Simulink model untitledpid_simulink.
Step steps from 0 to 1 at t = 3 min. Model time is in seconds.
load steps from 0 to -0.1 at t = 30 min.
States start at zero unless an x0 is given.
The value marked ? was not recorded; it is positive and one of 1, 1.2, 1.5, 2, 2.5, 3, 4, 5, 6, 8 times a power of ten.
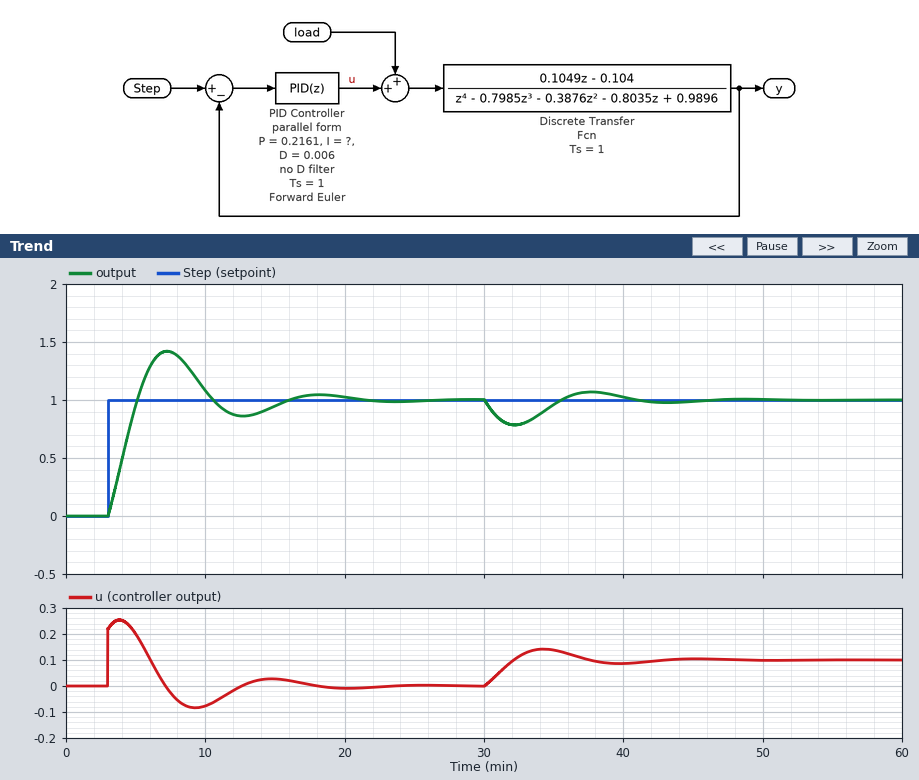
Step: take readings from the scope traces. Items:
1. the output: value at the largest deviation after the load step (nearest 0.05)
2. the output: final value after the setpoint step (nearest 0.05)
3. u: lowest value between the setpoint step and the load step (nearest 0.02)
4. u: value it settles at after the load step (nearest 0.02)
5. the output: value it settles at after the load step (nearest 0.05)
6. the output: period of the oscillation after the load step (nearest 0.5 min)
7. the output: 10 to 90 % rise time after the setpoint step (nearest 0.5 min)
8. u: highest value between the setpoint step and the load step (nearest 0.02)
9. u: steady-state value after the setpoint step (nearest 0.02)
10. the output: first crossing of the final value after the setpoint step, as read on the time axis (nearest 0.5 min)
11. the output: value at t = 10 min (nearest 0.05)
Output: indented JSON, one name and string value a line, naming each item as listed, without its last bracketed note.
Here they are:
{
  "the output: value at the largest deviation after the load step": "0.80",
  "the output: final value after the setpoint step": "1.00",
  "u: lowest value between the setpoint step and the load step": "-0.08",
  "u: value it settles at after the load step": "0.10",
  "the output: value it settles at after the load step": "1.00",
  "the output: period of the oscillation after the load step": "11.0 min",
  "the output: 10 to 90 % rise time after the setpoint step": "1.5 min",
  "u: highest value between the setpoint step and the load step": "0.26",
  "u: steady-state value after the setpoint step": "0.00",
  "the output: first crossing of the final value after the setpoint step, as read on the time axis": "5.0 min",
  "the output: value at t = 10 min": "1.10"
}
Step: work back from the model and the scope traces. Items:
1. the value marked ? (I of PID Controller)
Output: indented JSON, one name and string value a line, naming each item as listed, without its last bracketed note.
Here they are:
{
  "the value marked ?": "0.003"
}
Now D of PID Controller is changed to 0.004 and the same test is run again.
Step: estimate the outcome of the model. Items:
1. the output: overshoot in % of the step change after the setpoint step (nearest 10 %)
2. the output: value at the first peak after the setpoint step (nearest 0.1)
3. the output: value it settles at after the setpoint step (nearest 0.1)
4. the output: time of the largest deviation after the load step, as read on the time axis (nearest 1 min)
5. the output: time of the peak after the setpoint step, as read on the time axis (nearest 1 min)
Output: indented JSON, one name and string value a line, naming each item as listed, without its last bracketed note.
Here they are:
{
  "the output: overshoot in % of the step change after the setpoint step": "40 %",
  "the output: value at the first peak after the setpoint step": "1.4",
  "the output: value it settles at after the setpoint step": "1.0",
  "the output: time of the largest deviation after the load step, as read on the time axis": "32 min",
  "the output: time of the peak after the setpoint step, as read on the time axis": "7 min"
}
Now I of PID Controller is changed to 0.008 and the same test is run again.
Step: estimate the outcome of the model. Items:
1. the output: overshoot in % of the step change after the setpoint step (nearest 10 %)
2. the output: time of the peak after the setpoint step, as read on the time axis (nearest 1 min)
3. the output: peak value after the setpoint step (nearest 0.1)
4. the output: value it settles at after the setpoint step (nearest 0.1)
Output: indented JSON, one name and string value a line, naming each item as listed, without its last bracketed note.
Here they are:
{
  "the output: overshoot in % of the step change after the setpoint step": "60 %",
  "the output: time of the peak after the setpoint step, as read on the time axis": "6 min",
  "the output: peak value after the setpoint step": "1.6",
  "the output: value it settles at after the setpoint step": "1.0"
}
